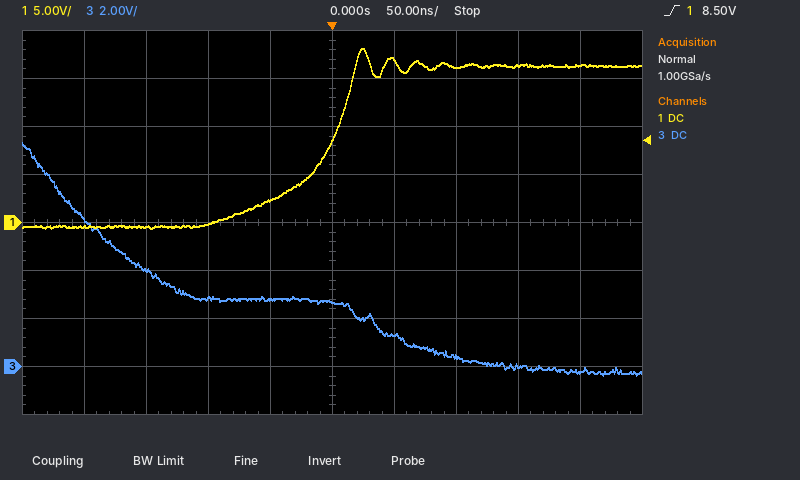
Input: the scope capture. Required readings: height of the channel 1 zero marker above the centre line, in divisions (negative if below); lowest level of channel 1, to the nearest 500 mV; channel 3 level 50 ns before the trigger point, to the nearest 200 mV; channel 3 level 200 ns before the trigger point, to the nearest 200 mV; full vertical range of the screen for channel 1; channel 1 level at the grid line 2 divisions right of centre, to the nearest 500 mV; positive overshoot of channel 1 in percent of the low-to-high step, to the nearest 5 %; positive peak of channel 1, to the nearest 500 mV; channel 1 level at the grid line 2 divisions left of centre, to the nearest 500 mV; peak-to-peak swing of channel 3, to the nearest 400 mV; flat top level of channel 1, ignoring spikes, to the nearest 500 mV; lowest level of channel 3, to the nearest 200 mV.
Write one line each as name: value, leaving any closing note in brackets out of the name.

height of the channel 1 zero marker above the centre line, in divisions: 0.0 div
lowest level of channel 1, to the nearest 500 mV: -500 mV
channel 3 level 50 ns before the trigger point, to the nearest 200 mV: 2.8 V
channel 3 level 200 ns before the trigger point, to the nearest 200 mV: 6.2 V
full vertical range of the screen for channel 1: 40 V
channel 1 level at the grid line 2 divisions right of centre, to the nearest 500 mV: 16.0 V
positive overshoot of channel 1 in percent of the low-to-high step, to the nearest 5 %: 10 %
positive peak of channel 1, to the nearest 500 mV: 18.0 V
channel 1 level at the grid line 2 divisions left of centre, to the nearest 500 mV: 0.0 V
peak-to-peak swing of channel 3, to the nearest 400 mV: 9.6 V
flat top level of channel 1, ignoring spikes, to the nearest 500 mV: 16.5 V
lowest level of channel 3, to the nearest 200 mV: -400 mV
